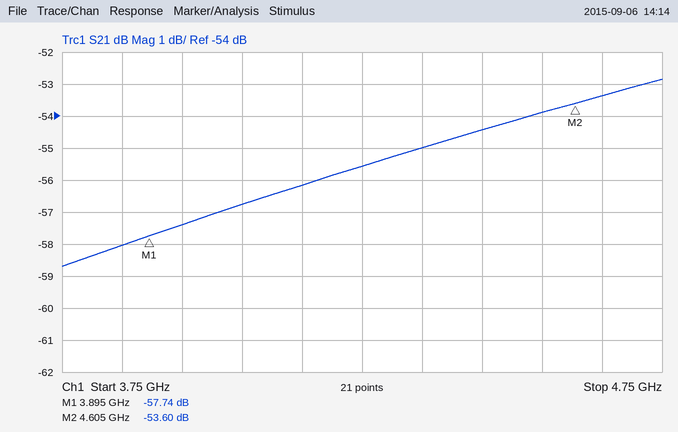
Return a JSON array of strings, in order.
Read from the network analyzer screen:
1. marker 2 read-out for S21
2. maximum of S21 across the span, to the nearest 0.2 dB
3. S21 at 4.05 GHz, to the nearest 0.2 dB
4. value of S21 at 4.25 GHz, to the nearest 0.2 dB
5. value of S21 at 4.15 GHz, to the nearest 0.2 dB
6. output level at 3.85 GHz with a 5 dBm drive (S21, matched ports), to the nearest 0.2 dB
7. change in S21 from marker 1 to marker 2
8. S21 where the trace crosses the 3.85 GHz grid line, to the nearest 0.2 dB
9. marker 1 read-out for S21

["-53.60 dB", "-52.8 dB", "-56.8 dB", "-55.6 dB", "-56.2 dB", "-53.0 dBm", "4.14 dB", "-58.0 dB", "-57.74 dB"]
